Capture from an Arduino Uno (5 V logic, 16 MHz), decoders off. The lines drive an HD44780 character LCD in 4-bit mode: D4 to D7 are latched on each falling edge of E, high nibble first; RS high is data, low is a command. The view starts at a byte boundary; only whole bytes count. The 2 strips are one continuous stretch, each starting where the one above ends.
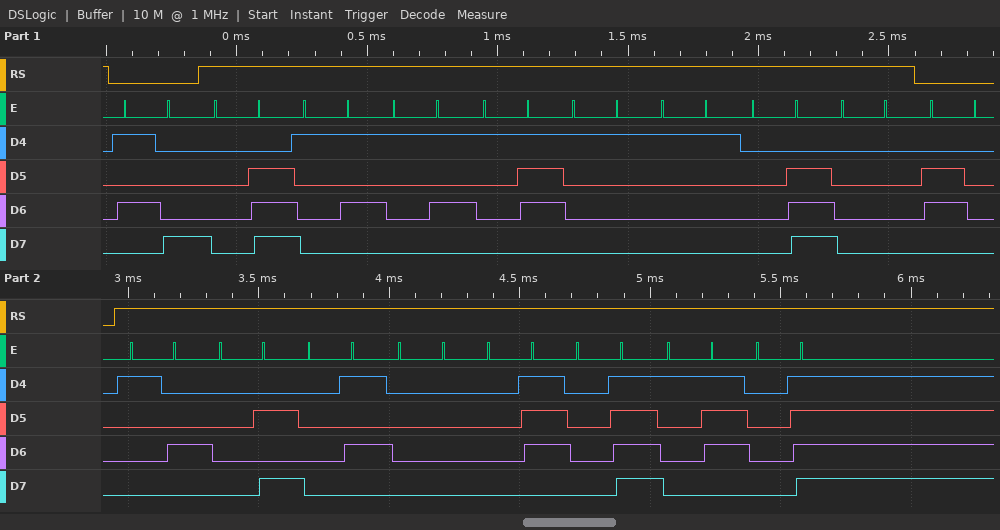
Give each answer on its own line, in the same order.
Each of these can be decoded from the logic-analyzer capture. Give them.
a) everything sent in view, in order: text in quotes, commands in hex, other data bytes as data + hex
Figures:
0x58 data 0E 15 15 17 11 11 0E 00 0x60 data 14 0A 05 00 07 0F 17 0F
